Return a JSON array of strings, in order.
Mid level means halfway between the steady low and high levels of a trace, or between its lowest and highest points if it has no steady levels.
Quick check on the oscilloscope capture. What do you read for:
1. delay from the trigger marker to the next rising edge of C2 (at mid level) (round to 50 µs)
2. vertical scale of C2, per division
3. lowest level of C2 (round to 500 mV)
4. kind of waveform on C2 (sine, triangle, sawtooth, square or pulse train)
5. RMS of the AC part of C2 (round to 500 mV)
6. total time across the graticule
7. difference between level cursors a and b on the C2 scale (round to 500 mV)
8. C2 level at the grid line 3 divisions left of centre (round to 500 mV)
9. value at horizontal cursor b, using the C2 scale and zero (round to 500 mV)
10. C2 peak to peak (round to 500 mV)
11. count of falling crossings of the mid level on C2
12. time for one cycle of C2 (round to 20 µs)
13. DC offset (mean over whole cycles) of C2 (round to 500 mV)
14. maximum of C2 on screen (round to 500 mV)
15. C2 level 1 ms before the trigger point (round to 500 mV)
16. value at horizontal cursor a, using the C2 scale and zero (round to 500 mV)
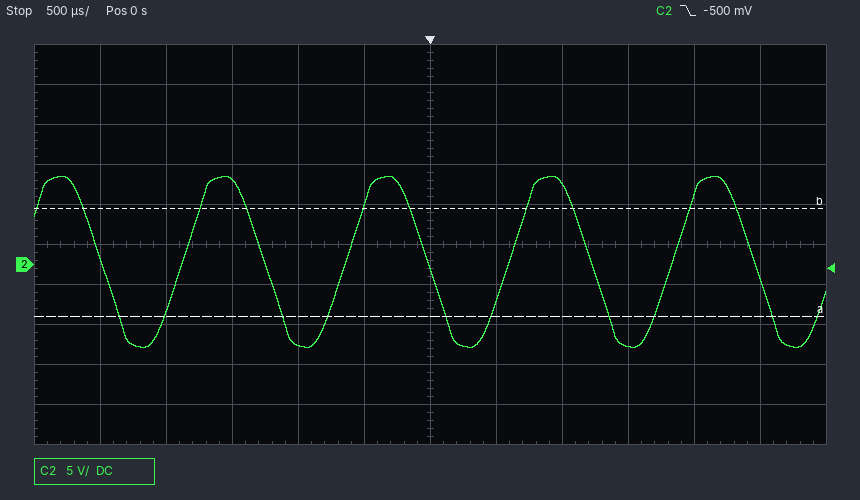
["600 µs", "5 V", "-10.5 V", "sine", "7.5 V", "6 ms", "13.5 V", "10.5 V", "7.0 V", "21.5 V", "5", "1.24 ms", "500 mV", "11.0 V", "-10.0 V", "-6.5 V"]
